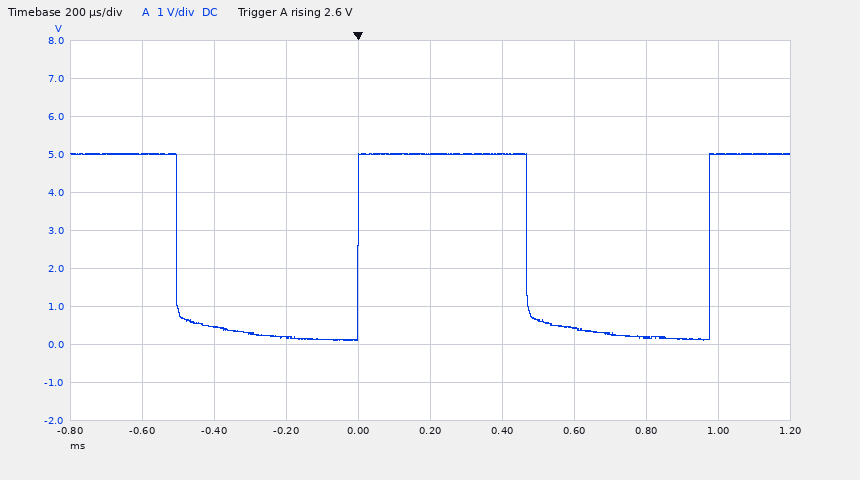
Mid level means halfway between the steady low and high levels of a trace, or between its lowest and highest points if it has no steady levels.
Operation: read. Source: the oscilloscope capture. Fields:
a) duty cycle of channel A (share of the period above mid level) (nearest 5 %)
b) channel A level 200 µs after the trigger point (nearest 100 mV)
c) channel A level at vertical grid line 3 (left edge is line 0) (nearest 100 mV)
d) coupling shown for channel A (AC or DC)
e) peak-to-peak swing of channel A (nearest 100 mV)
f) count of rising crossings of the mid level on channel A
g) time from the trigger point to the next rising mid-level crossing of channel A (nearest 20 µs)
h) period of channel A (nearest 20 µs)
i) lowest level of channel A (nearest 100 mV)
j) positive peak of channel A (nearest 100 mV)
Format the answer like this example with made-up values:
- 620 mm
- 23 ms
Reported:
- 50 %
- 5.0 V
- 200 mV
- DC
- 4.9 V
- 2
- 980 µs
- 980 µs
- 100 mV
- 5.0 V
